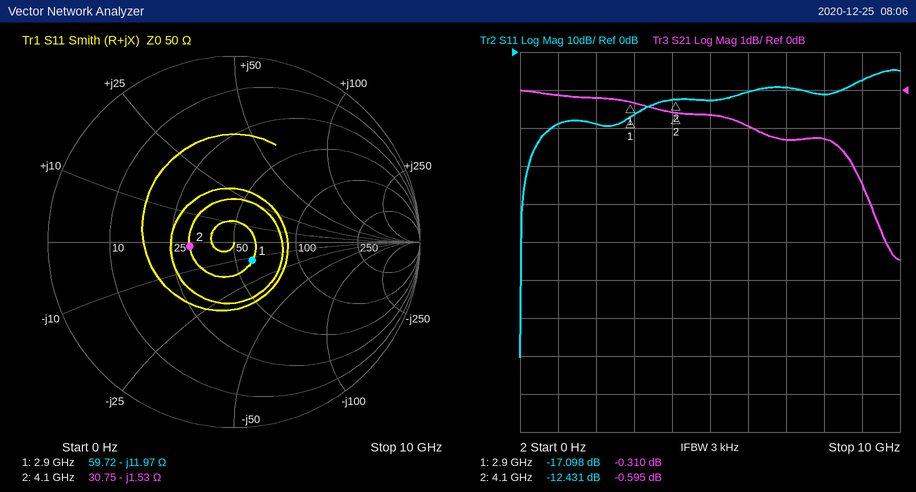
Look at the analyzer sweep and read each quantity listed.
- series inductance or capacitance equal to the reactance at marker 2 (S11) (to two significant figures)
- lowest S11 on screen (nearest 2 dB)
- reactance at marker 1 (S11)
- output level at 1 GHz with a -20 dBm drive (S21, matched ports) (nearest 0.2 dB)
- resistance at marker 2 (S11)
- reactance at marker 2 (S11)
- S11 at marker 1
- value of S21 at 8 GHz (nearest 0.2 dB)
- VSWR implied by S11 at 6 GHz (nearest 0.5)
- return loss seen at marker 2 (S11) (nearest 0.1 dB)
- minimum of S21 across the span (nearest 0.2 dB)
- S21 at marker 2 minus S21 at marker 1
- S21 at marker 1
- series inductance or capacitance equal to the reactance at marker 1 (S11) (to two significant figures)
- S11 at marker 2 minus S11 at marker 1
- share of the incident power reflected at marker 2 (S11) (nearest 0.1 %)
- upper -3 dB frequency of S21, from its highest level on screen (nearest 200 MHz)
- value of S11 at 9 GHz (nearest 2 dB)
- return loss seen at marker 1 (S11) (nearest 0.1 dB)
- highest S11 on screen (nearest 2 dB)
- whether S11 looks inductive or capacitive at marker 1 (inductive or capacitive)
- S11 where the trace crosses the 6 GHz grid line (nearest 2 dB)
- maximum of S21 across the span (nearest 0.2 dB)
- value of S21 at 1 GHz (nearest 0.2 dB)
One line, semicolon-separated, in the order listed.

25 pF; -80 dB; -11.97 Ω; -20.2 dBm; 30.75 Ω; -1.53 Ω; -17.098 dB; -1.2 dB; 2.0; 12.4 dB; -4.4 dB; -0.285 dB; -0.310 dB; 4.6 pF; 4.667 dB; 5.7 %; 9.2 GHz; -8 dB; 17.1 dB; -4 dB; capacitive; -10 dB; 0.0 dB; -0.2 dB
